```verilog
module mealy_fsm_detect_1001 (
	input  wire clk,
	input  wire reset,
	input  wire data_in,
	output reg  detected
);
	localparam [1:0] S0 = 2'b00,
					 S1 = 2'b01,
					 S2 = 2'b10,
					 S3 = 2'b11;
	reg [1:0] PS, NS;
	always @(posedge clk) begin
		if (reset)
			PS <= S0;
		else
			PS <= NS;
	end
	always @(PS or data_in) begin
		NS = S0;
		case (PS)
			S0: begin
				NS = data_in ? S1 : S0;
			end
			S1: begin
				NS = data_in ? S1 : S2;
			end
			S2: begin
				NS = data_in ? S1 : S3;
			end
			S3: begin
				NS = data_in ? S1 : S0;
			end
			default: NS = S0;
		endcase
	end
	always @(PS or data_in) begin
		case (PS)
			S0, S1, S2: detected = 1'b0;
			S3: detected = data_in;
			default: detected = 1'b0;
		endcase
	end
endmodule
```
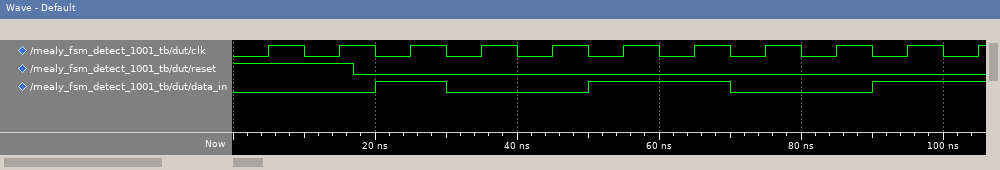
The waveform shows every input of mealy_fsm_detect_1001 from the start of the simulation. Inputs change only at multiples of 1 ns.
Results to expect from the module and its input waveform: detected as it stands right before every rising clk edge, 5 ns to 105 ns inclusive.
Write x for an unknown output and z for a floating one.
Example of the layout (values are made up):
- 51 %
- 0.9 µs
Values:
- 0 0 0 0 0 1 0 0 0 1 0
